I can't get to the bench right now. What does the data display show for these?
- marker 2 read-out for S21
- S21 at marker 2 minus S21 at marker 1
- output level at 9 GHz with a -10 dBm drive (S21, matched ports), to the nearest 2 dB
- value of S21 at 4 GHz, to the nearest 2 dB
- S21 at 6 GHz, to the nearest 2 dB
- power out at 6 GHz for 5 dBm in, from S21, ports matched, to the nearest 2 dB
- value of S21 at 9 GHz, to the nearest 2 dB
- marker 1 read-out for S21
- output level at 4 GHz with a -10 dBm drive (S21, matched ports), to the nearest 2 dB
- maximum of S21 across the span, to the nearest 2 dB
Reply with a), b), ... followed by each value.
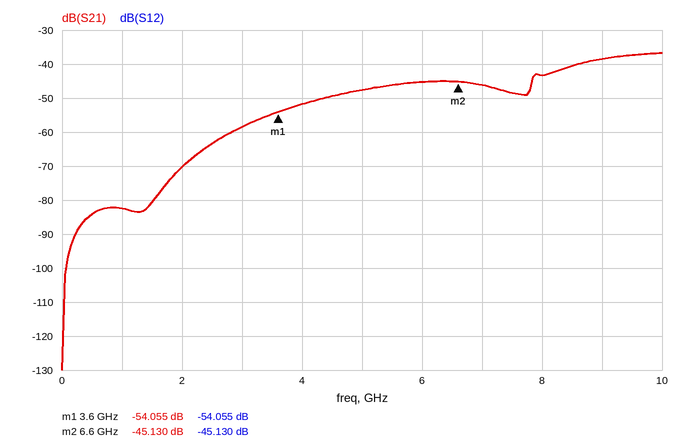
a) -45.130 dB
b) 8.925 dB
c) -48 dBm
d) -52 dB
e) -46 dB
f) -40 dBm
g) -38 dB
h) -54.055 dB
i) -62 dBm
j) -36 dB
